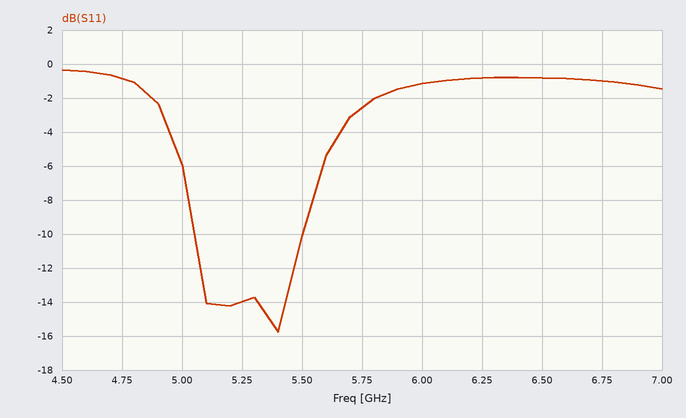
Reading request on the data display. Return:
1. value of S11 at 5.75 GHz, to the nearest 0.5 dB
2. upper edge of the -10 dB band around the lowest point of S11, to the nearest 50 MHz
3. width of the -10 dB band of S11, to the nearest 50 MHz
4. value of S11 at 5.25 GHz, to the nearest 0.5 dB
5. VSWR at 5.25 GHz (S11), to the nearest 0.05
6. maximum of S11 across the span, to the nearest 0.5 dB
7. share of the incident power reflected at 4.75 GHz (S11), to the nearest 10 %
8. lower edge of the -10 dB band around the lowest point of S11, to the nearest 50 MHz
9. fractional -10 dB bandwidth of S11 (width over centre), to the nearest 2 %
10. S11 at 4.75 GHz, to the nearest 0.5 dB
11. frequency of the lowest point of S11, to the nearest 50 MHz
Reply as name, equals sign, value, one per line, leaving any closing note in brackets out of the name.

value of S11 at 5.75 GHz, to the nearest 0.5 dB = -2.5 dB
upper edge of the -10 dB band around the lowest point of S11, to the nearest 50 MHz = 5.50 GHz
width of the -10 dB band of S11, to the nearest 50 MHz = 450 MHz
value of S11 at 5.25 GHz, to the nearest 0.5 dB = -14.0 dB
VSWR at 5.25 GHz (S11), to the nearest 0.05 = 1.50
maximum of S11 across the span, to the nearest 0.5 dB = -0.5 dB
share of the incident power reflected at 4.75 GHz (S11), to the nearest 10 % = 80 %
lower edge of the -10 dB band around the lowest point of S11, to the nearest 50 MHz = 5.05 GHz
fractional -10 dB bandwidth of S11 (width over centre), to the nearest 2 % = 8 %
S11 at 4.75 GHz, to the nearest 0.5 dB = -1.0 dB
frequency of the lowest point of S11, to the nearest 50 MHz = 5.40 GHz
